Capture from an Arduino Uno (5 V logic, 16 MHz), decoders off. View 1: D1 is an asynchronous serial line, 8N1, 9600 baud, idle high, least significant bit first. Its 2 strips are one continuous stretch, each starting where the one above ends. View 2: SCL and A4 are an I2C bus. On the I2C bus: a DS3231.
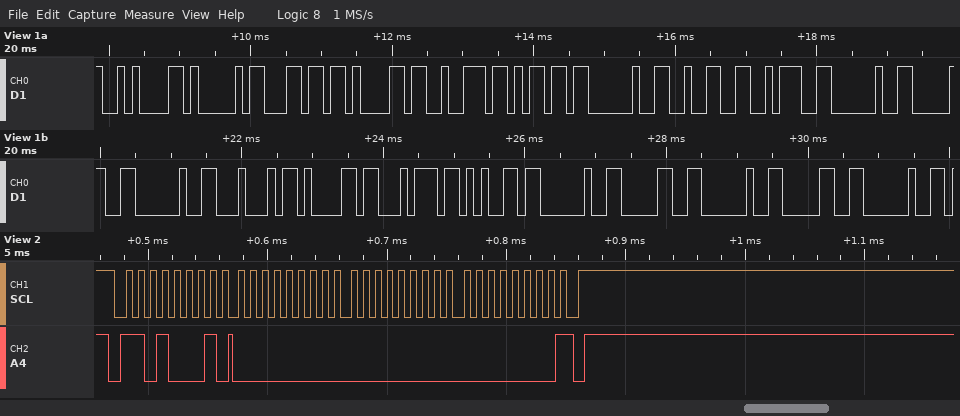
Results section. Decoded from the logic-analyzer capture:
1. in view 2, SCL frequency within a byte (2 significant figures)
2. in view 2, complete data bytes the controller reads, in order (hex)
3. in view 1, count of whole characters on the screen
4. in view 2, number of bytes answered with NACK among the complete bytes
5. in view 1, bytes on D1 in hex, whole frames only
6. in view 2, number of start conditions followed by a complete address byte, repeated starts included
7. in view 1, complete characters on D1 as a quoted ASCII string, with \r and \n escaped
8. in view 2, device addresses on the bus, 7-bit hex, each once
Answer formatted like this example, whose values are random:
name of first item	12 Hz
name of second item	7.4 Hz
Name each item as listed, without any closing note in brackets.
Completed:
in view 2, SCL frequency within a byte	100 kHz
in view 2, complete data bytes the controller reads, in order	00 00 00
in view 1, count of whole characters on the screen	21
in view 2, number of bytes answered with NACK among the complete bytes	1
in view 1, bytes on D1 in hex, whole frames only	0x0A 0x41 0x6C 0x61 0x72 0x6D 0x20 0x32 0x3A 0x20 0x30 0x20 0x44 0x61 0x74 0x65 0x20 0x30 0x20 0x30 0x20
in view 2, number of start conditions followed by a complete address byte, repeated starts included	1
in view 1, complete characters on D1 as a quoted ASCII string, with \r and \n escaped	"\nAlarm 2: 0 Date 0 0 "
in view 2, device addresses on the bus, 7-bit hex, each once	0x68
